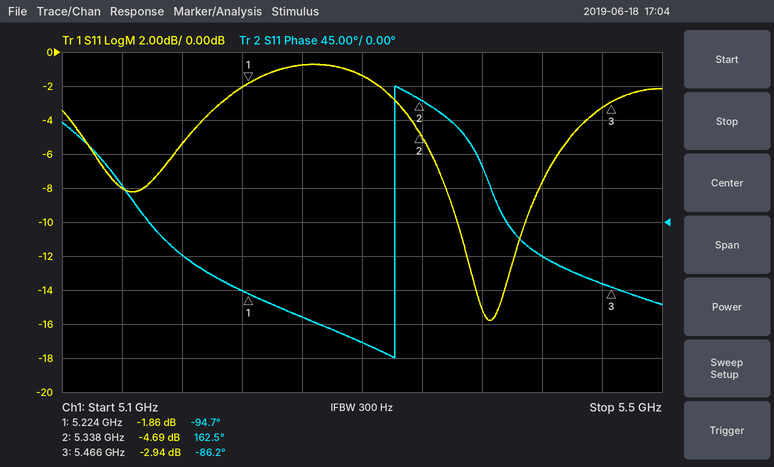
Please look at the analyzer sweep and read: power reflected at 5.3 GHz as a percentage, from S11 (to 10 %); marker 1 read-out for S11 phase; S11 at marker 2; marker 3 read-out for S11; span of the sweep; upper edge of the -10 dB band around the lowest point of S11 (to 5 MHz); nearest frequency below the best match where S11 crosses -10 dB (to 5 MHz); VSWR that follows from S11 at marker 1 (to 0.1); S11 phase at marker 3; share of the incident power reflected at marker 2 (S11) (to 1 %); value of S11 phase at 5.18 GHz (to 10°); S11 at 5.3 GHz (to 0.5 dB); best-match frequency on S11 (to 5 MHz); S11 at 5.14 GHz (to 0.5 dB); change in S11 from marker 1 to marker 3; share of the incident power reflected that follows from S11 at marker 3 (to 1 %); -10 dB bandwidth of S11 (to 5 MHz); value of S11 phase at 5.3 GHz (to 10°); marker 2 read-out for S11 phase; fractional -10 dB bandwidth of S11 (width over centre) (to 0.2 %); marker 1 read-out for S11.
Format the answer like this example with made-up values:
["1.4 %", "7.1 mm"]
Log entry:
["70 %", "-94.7°", "-4.69 dB", "-2.94 dB", "400 MHz", "5.410 GHz", "5.365 GHz", "9.4", "-86.2°", "34 %", "-40°", "-1.5 dB", "5.385 GHz", "-8.0 dB", "-1.08 dB", "51 %", "45 MHz", "-160°", "162.5°", "0.8 %", "-1.86 dB"]
